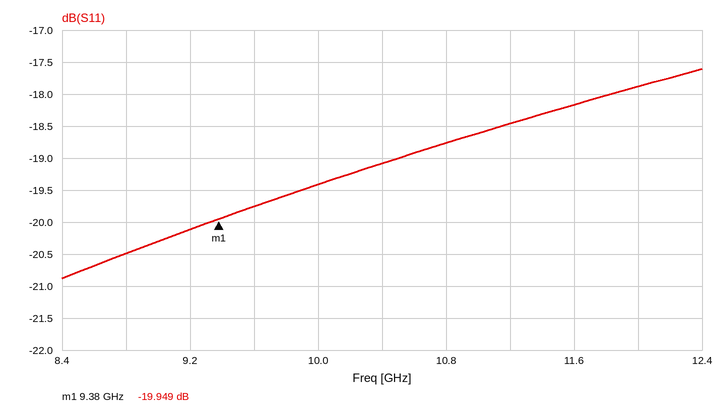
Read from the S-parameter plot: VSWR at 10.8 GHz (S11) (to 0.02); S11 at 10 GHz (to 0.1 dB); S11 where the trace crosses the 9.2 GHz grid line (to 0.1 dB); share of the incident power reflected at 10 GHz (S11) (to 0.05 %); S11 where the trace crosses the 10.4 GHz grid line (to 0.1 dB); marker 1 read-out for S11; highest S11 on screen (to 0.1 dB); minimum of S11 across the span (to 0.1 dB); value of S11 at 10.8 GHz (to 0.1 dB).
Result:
1.26
-19.4 dB
-20.1 dB
1.15 %
-19.1 dB
-19.949 dB
-17.6 dB
-20.9 dB
-18.8 dB
